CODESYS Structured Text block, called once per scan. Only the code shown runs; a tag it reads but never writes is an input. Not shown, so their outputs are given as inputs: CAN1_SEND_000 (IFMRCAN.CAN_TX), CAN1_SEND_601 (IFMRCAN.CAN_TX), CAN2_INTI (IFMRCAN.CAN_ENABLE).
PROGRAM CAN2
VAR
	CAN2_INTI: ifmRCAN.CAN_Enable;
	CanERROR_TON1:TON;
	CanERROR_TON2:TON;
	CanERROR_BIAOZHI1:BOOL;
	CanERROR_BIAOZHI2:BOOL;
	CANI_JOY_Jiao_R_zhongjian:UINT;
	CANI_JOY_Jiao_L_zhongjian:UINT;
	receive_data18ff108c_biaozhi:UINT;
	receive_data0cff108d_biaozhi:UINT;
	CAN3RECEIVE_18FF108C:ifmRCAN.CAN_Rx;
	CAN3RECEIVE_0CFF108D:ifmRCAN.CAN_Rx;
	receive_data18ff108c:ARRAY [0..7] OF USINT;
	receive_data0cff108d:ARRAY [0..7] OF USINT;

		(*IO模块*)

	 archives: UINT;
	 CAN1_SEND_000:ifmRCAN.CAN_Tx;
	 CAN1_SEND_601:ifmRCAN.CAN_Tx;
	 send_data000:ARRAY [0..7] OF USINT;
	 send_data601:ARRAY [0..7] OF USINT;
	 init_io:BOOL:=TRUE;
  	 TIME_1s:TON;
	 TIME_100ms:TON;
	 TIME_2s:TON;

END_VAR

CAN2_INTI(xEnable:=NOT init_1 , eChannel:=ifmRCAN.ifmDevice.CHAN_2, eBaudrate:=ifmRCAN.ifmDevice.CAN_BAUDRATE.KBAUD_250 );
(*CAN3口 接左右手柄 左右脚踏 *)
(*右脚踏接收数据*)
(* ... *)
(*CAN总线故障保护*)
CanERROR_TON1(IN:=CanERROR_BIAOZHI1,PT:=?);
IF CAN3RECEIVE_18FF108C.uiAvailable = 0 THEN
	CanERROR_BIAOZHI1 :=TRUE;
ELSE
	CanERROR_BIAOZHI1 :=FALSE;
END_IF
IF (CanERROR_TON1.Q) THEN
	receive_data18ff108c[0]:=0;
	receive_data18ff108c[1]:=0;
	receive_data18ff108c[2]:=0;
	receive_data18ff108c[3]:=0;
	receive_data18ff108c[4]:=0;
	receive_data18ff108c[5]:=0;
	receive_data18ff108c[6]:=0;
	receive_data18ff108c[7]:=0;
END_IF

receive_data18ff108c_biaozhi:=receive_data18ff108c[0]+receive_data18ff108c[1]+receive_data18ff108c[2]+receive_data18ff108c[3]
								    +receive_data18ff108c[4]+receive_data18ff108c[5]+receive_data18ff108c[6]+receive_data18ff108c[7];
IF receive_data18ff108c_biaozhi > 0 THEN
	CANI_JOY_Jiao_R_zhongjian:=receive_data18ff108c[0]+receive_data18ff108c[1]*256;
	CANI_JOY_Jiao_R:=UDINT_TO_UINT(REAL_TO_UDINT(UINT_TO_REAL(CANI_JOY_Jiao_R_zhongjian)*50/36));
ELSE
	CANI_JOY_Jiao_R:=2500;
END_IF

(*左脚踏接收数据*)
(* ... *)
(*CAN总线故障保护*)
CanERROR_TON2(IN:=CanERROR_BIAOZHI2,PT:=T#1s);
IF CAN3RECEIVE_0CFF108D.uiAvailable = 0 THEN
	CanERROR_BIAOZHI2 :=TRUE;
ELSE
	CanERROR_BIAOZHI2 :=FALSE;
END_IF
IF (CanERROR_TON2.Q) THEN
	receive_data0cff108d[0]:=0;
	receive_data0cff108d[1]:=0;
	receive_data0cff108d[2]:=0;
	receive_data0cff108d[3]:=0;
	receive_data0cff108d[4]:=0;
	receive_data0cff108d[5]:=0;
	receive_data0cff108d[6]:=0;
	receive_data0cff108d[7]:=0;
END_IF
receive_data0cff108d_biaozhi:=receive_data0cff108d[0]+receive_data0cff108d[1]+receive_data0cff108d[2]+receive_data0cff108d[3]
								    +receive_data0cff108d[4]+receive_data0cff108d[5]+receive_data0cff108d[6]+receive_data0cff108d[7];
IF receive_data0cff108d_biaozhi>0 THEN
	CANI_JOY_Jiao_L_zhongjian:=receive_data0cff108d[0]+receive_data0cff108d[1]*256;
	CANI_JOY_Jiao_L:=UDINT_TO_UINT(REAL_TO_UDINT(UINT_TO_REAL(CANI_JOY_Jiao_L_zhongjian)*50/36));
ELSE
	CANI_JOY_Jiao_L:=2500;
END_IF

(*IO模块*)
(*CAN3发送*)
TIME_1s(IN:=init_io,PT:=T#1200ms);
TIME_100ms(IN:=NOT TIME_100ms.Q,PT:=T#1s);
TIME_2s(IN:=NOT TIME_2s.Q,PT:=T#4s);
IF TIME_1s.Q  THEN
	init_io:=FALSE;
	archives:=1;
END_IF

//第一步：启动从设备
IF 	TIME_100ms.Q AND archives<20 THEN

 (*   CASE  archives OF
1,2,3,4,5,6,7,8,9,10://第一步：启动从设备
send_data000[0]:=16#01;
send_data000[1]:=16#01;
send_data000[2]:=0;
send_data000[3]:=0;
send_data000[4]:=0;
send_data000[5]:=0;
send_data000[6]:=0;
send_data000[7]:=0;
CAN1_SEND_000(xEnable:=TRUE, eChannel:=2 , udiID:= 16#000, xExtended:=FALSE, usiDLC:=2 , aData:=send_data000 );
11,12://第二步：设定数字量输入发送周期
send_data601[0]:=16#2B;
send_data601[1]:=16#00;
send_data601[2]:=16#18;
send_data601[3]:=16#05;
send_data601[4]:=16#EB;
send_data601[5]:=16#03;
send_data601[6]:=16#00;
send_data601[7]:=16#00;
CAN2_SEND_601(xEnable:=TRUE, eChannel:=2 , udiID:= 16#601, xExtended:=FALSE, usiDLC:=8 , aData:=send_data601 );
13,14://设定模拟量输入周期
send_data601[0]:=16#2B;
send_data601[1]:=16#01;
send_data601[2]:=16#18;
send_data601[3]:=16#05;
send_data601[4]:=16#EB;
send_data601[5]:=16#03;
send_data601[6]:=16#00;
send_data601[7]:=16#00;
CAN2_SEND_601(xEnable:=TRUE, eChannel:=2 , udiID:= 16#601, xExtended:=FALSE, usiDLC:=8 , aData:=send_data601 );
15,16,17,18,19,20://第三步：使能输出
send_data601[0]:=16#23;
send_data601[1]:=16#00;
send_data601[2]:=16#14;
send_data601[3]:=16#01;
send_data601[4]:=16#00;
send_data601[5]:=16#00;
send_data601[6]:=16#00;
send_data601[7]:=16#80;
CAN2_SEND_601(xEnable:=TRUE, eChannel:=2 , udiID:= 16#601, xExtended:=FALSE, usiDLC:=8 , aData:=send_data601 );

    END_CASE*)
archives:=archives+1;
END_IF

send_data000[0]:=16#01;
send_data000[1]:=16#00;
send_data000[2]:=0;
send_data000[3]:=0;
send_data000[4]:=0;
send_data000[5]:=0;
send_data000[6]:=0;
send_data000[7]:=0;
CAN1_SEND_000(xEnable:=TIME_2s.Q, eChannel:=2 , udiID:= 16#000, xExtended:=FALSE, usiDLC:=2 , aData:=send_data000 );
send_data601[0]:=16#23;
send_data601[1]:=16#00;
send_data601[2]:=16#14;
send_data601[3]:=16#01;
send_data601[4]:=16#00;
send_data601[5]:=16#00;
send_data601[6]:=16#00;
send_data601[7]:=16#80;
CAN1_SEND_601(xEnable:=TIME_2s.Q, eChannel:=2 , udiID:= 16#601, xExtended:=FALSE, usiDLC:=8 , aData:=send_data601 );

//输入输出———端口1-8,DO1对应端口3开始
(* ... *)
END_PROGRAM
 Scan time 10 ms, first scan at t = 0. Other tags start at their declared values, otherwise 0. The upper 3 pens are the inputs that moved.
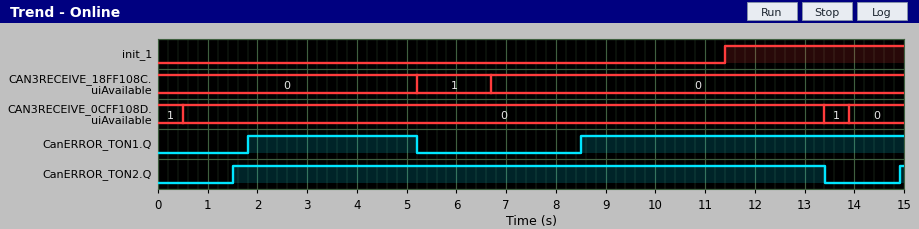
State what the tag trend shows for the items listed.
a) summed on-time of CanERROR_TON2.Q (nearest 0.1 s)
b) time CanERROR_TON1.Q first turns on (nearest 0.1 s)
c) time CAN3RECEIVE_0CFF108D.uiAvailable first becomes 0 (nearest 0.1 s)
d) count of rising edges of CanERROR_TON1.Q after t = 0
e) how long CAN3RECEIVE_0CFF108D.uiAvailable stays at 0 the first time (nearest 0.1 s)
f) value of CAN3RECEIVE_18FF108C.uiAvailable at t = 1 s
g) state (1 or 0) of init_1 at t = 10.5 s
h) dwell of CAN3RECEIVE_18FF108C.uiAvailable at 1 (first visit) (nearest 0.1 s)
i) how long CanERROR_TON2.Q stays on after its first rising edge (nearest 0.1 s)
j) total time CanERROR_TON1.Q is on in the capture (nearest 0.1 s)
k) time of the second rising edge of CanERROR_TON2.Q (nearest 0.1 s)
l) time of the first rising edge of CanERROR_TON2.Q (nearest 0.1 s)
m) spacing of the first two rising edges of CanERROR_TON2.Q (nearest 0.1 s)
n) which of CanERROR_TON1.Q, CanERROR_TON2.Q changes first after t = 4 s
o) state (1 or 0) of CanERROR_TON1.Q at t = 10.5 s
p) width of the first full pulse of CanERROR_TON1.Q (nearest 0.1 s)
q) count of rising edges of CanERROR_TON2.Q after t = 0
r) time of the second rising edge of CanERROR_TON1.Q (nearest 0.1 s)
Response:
12.0 s
1.8 s
0.5 s
2
12.9 s
0
0
1.5 s
11.9 s
9.9 s
14.9 s
1.5 s
13.4 s
CanERROR_TON1.Q
1
3.4 s
2
8.5 s
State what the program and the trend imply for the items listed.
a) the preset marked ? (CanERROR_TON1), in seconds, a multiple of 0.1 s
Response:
1.8 s
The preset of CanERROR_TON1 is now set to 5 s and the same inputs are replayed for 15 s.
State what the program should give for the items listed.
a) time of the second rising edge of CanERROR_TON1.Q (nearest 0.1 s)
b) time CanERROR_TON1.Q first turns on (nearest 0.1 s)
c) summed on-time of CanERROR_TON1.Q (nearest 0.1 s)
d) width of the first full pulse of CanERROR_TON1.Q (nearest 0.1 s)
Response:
11.7 s
5.0 s
3.5 s
0.2 s
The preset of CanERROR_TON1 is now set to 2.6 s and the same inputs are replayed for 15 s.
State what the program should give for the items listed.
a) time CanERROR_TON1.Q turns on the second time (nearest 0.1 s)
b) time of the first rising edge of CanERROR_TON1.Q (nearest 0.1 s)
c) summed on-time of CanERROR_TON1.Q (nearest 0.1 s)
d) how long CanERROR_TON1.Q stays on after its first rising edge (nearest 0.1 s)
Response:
9.3 s
2.6 s
8.3 s
2.6 s
